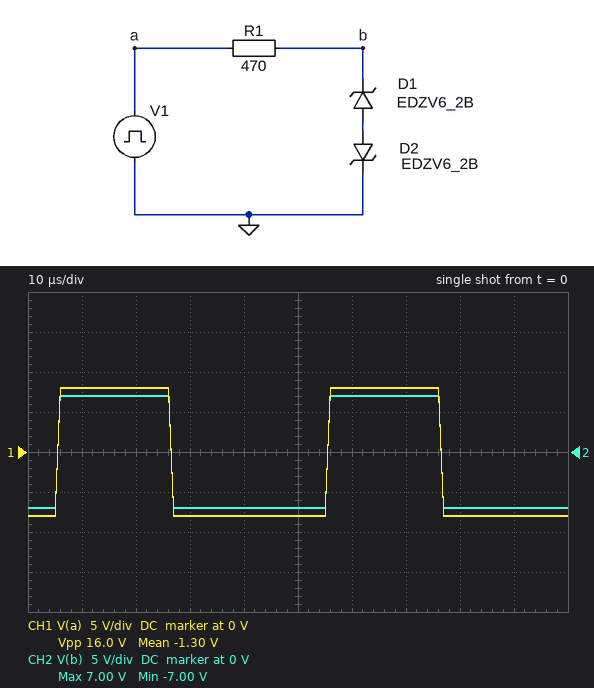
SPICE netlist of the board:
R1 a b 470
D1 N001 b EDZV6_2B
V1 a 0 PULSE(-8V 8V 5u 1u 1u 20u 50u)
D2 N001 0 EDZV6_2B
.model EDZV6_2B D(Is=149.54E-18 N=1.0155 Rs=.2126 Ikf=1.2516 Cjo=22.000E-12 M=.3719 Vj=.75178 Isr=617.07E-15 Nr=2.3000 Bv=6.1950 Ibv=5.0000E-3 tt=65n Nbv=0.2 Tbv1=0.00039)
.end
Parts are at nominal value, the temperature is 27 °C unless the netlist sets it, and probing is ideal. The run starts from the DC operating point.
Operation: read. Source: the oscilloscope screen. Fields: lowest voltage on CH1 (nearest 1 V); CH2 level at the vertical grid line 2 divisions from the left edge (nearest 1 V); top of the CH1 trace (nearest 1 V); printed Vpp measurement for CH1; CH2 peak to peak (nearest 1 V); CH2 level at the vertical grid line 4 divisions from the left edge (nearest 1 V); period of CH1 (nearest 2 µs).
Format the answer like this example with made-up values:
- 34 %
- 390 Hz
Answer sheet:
- -8 V
- 7 V
- 8 V
- 16.0 V
- 14 V
- -7 V
- 50 µs
